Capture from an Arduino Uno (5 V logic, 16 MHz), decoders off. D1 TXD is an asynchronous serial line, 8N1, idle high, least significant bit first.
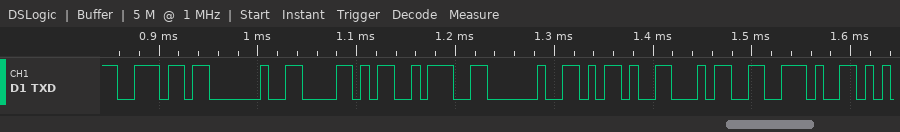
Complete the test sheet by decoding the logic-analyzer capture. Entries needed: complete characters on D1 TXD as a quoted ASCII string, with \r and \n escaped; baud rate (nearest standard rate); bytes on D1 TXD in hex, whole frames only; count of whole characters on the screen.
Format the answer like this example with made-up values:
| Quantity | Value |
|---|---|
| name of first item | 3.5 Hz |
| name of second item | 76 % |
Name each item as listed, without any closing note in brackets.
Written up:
| Quantity | Value |
|---|---|
| complete characters on D1 TXD as a quoted ASCII string, with \r and \n escaped | "n X: -4." |
| baud rate | 115200 baud |
| bytes on D1 TXD in hex, whole frames only | 0x6E 0x20 0x58 0x3A 0x20 0x2D 0x34 0x2E |
| count of whole characters on the screen | 8 |
